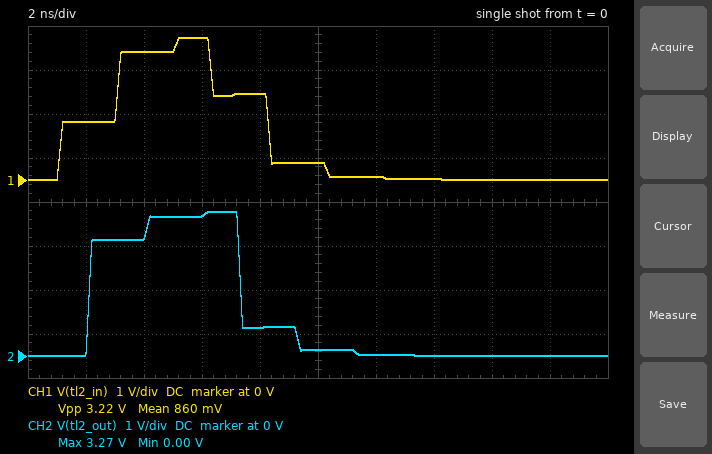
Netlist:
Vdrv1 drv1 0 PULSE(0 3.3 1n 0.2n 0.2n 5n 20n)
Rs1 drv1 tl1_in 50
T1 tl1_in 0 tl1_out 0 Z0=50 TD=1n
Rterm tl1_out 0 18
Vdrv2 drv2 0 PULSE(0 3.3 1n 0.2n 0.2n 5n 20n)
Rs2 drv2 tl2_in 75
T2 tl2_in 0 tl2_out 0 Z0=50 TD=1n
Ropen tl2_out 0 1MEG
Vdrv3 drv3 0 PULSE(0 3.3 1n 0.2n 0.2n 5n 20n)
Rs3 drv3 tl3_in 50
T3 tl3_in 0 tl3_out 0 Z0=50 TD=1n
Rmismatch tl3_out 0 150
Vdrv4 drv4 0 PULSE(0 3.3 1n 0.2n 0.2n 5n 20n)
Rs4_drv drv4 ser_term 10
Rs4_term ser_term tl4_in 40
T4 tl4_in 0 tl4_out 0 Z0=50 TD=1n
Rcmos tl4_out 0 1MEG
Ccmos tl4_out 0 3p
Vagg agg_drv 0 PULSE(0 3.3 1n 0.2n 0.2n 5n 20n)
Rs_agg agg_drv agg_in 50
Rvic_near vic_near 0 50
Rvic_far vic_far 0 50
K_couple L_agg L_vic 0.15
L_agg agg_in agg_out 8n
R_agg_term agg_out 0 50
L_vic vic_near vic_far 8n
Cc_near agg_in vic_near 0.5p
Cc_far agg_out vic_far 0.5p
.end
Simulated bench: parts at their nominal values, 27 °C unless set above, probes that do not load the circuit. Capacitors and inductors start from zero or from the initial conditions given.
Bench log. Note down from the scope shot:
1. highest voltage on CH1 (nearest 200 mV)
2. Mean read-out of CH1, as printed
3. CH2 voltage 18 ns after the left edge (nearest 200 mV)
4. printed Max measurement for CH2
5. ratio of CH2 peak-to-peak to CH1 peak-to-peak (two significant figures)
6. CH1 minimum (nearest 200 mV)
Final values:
3.2 V
860 mV
0 V
3.27 V
1.0
0 V
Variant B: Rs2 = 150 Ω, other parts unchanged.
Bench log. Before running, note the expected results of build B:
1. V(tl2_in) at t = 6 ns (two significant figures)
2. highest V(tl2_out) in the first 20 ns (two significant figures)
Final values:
2.7 V
2.9 V
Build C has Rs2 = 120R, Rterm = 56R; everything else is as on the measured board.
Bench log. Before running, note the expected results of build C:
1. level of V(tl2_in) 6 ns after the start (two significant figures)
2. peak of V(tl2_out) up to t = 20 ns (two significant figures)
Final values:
2.9 V
3.1 V
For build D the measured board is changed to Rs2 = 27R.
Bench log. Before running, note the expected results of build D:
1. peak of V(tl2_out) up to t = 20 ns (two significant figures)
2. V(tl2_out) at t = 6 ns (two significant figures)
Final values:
4.3 V
3.0 V
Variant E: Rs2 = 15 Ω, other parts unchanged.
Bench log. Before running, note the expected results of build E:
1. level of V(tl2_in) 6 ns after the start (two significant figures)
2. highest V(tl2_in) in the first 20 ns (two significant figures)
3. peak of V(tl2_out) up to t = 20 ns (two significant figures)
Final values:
3.1 V
3.7 V
5.1 V
